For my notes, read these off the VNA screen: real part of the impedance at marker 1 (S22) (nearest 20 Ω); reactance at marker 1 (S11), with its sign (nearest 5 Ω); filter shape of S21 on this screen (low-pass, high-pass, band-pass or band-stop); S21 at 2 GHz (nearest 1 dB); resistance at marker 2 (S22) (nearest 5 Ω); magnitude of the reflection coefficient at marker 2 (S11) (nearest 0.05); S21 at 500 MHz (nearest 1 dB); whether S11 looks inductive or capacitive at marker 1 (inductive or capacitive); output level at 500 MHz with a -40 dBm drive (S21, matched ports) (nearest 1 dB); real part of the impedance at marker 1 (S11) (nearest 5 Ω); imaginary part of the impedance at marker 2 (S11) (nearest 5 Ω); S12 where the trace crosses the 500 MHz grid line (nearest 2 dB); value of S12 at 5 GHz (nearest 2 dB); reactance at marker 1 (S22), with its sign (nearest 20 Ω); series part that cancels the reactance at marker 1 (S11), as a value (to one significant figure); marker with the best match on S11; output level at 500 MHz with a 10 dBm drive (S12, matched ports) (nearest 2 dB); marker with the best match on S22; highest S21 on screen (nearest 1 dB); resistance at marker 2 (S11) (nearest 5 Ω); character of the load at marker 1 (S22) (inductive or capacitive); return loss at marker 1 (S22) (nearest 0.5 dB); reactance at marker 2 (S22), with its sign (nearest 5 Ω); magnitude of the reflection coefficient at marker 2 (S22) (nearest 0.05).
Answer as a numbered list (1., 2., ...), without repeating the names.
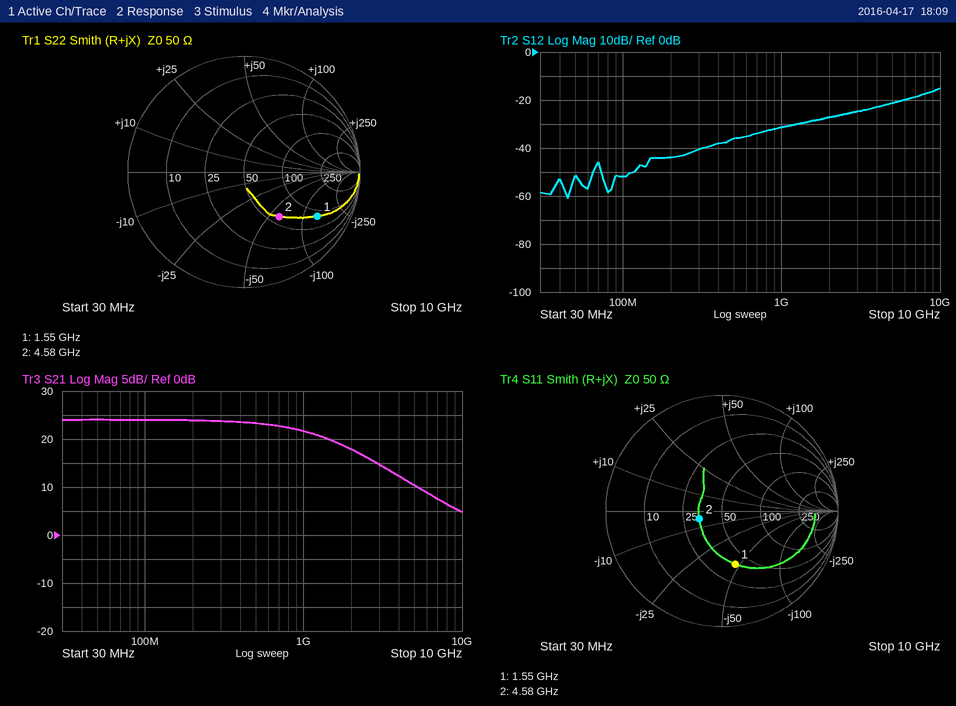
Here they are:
1. 80 Ω
2. -45 Ω
3. low-pass
4. 18 dB
5. 60 Ω
6. 0.20
7. 23 dB
8. capacitive
9. -17 dBm
10. 40 Ω
11. -5 Ω
12. -36 dB
13. -22 dB
14. -140 Ω
15. 5 nH
16. marker 2
17. -26 dBm
18. marker 2
19. 24 dB
20. 35 Ω
21. capacitive
22. 2.5 dB
23. -60 Ω
24. 0.50
